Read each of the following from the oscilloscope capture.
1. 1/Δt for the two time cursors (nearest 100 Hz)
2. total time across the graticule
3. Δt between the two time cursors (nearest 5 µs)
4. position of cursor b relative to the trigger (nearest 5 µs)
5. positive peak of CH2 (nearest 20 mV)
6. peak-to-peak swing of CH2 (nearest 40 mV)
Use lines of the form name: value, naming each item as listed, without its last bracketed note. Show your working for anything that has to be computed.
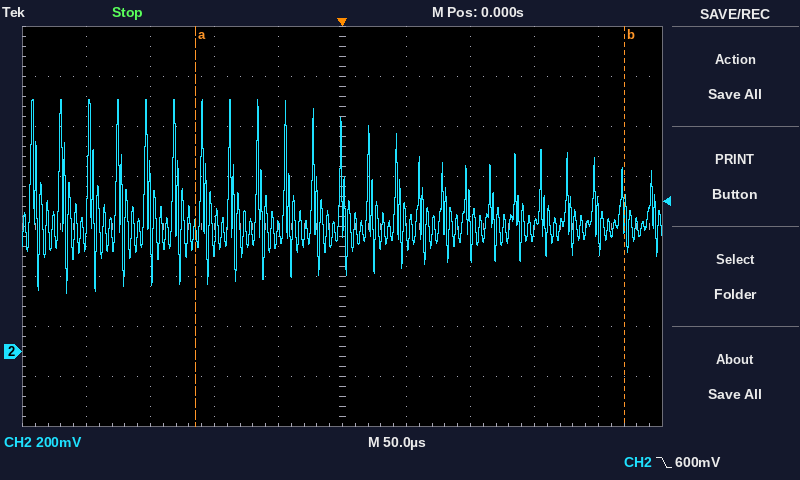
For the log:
1/Δt for the two time cursors: 1 / 335 µs ≈ 3.0 kHz
total time across the graticule: 500 µs
Δt between the two time cursors: 335 µs
position of cursor b relative to the trigger: +220 µs
positive peak of CH2: 1.00 V
peak-to-peak swing of CH2: 760 mV
